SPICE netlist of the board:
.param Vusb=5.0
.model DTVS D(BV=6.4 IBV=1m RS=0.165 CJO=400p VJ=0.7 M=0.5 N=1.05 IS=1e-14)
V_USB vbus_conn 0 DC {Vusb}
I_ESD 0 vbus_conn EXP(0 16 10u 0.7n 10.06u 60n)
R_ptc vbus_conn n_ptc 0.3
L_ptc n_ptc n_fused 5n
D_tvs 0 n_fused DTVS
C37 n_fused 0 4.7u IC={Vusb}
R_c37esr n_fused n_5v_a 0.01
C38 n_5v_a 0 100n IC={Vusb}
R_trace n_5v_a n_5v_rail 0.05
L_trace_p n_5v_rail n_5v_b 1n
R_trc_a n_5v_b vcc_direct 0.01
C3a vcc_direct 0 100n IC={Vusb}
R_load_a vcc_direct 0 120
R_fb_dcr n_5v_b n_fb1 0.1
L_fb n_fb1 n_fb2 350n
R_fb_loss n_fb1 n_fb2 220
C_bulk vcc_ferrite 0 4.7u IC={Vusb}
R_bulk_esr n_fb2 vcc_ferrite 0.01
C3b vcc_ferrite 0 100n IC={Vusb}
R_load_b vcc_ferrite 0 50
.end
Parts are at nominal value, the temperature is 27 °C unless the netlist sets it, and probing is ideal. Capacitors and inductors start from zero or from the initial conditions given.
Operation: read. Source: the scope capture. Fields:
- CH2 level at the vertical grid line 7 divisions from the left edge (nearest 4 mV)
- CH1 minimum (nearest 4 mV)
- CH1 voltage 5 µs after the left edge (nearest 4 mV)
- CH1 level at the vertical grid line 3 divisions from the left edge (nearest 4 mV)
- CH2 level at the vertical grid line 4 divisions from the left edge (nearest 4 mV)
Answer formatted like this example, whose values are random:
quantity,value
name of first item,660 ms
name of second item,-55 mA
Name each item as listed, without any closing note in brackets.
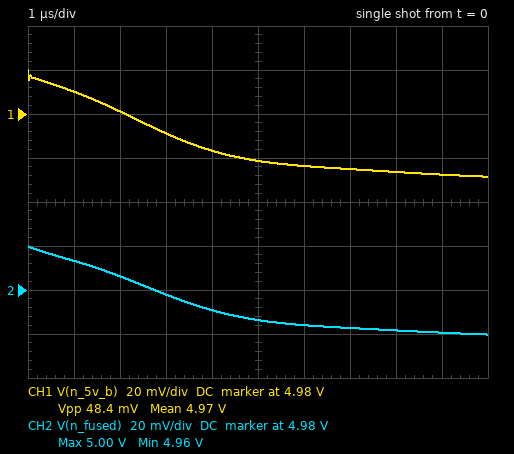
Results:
quantity,value
CH2 level at the vertical grid line 7 divisions from the left edge,4.964 V
CH1 minimum,4.952 V
CH1 voltage 5 µs after the left edge,4.960 V
CH1 level at the vertical grid line 3 divisions from the left edge,4.972 V
CH2 level at the vertical grid line 4 divisions from the left edge,4.972 V
